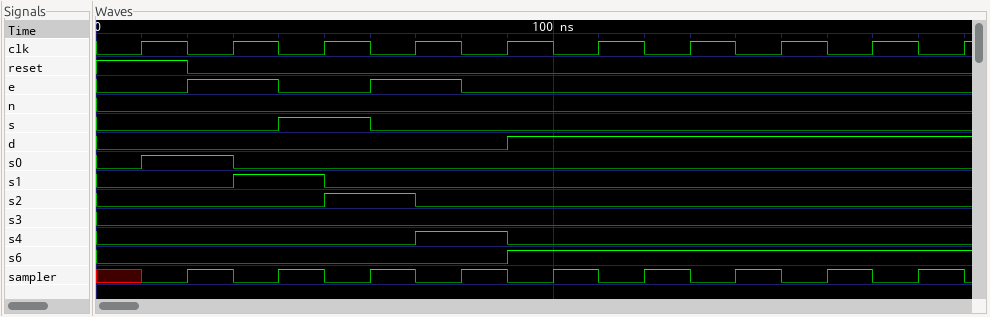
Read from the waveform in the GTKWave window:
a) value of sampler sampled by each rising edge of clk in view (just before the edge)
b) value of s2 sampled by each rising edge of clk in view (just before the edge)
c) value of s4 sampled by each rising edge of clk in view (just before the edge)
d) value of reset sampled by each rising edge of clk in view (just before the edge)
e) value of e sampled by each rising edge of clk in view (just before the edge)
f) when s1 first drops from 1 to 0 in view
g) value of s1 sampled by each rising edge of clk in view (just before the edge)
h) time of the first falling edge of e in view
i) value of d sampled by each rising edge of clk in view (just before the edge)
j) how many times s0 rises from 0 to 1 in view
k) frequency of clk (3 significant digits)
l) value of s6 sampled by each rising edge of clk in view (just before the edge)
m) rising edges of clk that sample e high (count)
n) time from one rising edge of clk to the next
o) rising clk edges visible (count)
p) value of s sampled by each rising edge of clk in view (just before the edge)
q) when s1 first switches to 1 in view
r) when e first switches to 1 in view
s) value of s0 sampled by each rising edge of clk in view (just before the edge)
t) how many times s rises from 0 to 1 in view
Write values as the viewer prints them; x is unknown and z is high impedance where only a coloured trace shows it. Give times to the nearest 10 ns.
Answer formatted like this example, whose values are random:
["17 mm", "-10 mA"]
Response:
["x 1 1 1 1 1 1 1 1 1", "0 0 0 1 0 0 0 0 0 0", "0 0 0 0 1 0 0 0 0 0", "1 0 0 0 0 0 0 0 0 0", "0 1 0 1 0 0 0 0 0 0", "50 ns", "0 0 1 0 0 0 0 0 0 0", "40 ns", "0 0 0 0 0 1 1 1 1 1", "1", "50.0 MHz", "0 0 0 0 0 1 1 1 1 1", "2", "20 ns", "10", "0 0 1 0 0 0 0 0 0 0", "30 ns", "20 ns", "0 1 0 0 0 0 0 0 0 0", "1"]
